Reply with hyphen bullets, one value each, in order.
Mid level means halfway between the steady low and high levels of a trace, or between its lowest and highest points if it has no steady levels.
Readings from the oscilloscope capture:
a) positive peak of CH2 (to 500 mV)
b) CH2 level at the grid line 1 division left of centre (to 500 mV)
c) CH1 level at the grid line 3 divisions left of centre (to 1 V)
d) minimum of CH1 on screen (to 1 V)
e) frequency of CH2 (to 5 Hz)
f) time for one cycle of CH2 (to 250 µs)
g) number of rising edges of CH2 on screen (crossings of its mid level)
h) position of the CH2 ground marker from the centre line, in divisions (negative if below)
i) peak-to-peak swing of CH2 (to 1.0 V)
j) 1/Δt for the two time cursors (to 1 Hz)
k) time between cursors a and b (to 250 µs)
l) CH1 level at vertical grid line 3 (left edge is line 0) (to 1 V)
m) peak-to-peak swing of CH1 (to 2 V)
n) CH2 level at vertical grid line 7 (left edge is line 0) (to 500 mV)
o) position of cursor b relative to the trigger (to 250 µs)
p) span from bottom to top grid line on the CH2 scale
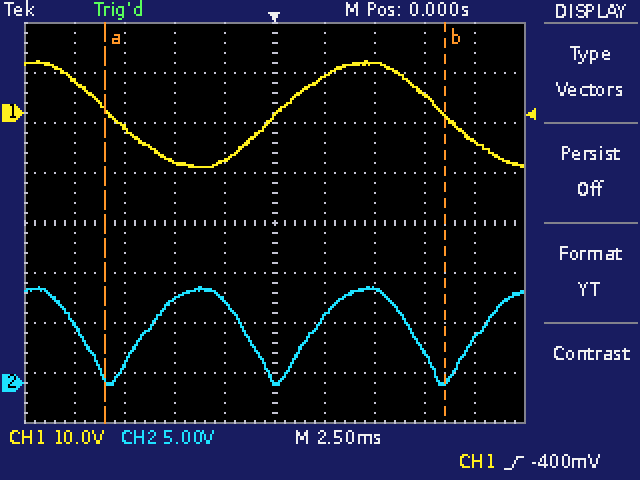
- 9.5 V
- 8.0 V
- -3 V
- -11 V
- 120 Hz
- 8.25 ms
- 3
- -3.2 div
- 10.0 V
- 59 Hz
- 17.00 ms
- -10 V
- 22 V
- 9.5 V
- +8.50 ms
- 40 V
